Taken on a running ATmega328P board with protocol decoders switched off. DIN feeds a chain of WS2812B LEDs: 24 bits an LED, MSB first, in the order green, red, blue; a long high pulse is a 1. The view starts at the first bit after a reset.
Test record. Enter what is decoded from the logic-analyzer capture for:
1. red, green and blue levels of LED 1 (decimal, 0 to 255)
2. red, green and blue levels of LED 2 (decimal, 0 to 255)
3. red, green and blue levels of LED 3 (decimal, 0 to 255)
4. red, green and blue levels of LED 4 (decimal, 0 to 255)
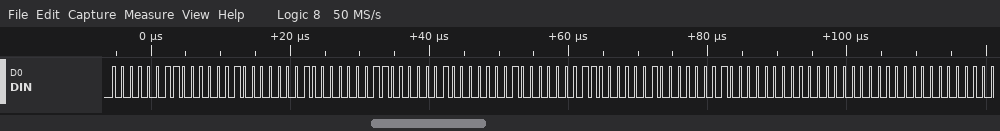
2, 3, 2
2, 3, 2
2, 3, 2
0, 0, 0
